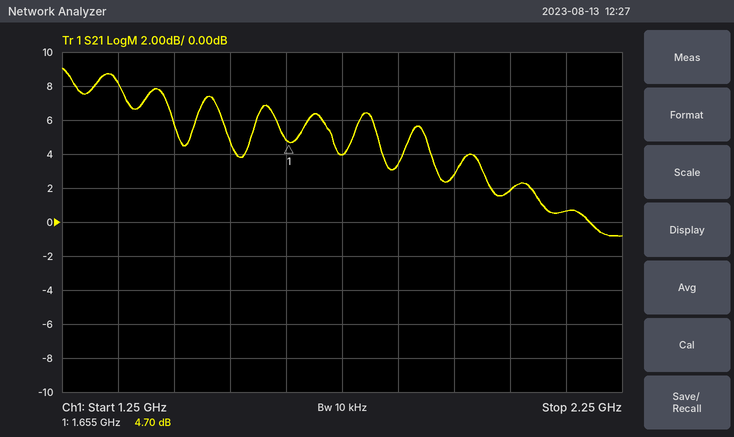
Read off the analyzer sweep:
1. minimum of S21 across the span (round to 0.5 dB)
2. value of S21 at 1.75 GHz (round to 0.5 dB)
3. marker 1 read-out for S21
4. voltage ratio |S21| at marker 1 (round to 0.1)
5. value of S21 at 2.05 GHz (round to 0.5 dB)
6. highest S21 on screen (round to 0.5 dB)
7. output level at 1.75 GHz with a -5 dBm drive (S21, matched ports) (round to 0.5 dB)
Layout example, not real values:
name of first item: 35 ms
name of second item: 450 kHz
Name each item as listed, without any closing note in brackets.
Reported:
minimum of S21 across the span: -1.0 dB
value of S21 at 1.75 GHz: 4.0 dB
marker 1 read-out for S21: 4.70 dB
voltage ratio |S21| at marker 1: 1.7
value of S21 at 2.05 GHz: 2.0 dB
highest S21 on screen: 9.0 dB
output level at 1.75 GHz with a -5 dBm drive (S21, matched ports): -1.0 dBm
